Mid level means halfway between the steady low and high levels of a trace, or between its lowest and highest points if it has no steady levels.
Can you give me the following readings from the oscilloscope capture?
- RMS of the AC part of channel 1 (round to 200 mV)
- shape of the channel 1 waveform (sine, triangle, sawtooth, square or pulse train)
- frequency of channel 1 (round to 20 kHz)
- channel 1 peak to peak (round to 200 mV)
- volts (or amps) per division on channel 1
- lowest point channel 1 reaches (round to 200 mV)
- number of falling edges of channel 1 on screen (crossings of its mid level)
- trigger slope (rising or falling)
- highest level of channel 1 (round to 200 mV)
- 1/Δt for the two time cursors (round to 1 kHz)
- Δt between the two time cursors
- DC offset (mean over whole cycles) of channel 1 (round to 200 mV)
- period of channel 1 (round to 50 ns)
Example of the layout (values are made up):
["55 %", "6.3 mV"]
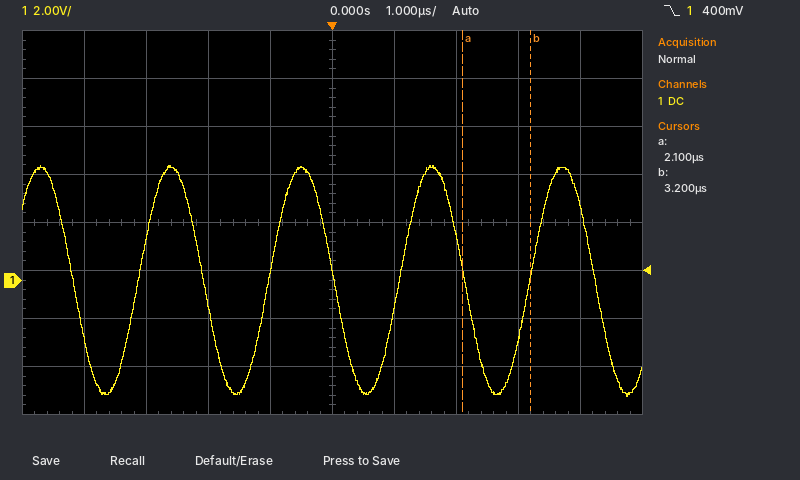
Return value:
["3.4 V", "sine", "480 kHz", "9.6 V", "2 V", "-4.8 V", "5", "falling", "4.8 V", "909 kHz", "1.1 µs", "0.0 V", "2.10 µs"]
